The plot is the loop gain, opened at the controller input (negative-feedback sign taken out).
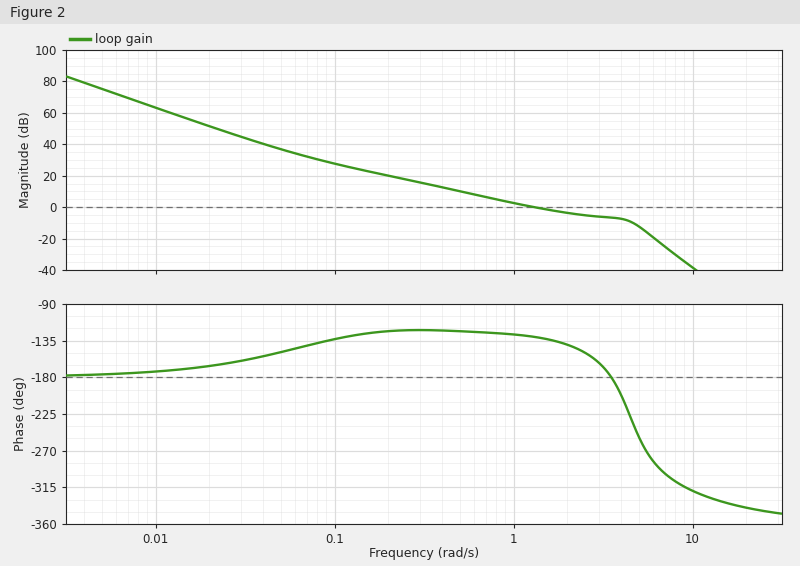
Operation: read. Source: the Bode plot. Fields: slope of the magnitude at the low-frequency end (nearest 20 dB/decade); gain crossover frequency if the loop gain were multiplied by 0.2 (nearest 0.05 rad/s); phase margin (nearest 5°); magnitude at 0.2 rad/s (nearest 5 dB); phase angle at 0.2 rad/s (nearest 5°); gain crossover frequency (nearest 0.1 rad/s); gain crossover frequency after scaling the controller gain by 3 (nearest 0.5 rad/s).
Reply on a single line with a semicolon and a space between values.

-40 dB/decade; 0.35 rad/s; 50°; 20 dB; -125°; 1.3 rad/s; 4.5 rad/s
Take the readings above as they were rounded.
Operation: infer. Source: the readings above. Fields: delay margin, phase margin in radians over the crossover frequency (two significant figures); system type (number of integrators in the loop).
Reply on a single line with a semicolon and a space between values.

0.67 s; 2
